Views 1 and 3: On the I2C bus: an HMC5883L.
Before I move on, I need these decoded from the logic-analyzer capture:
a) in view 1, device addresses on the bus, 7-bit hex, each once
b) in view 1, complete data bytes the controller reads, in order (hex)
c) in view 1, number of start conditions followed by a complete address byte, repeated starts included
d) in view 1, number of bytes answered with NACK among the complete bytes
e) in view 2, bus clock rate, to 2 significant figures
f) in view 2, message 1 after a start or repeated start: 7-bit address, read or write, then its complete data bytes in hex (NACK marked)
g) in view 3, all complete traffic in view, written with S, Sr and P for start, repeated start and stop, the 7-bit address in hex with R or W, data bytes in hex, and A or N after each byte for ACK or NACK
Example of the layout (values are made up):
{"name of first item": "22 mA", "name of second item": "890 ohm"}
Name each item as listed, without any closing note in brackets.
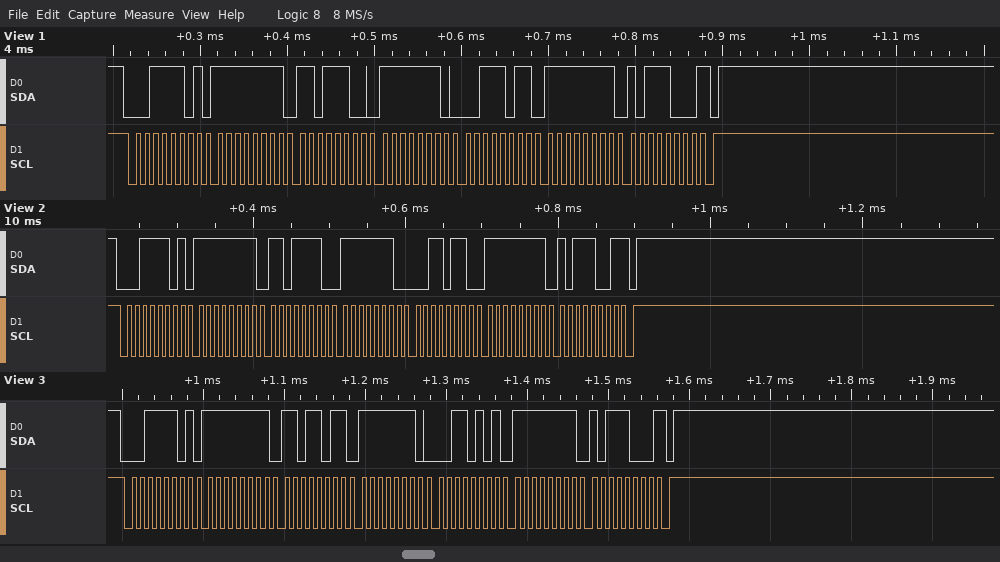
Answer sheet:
{"in view 1, device addresses on the bus, 7-bit hex, each once": "0x1E", "in view 1, complete data bytes the controller reads, in order": "FF DC FE 3B FF B8", "in view 1, number of start conditions followed by a complete address byte, repeated starts included": "1", "in view 1, number of bytes answered with NACK among the complete bytes": "1", "in view 2, bus clock rate, to 2 significant figures": "100 kHz", "in view 2, message 1 after a start or repeated start: 7-bit address, read or write, then its complete data bytes in hex": "0x1E read: FF DE FE 36 FF B9 NACK", "in view 3, all complete traffic in view, written with S, Sr and P for start, repeated start and stop, the 7-bit address in hex with R or W, data bytes in hex, and A or N after each byte for ACK or NACK": "S 1ER A FF A DB A FE A 35 A FF A B8 N P"}
